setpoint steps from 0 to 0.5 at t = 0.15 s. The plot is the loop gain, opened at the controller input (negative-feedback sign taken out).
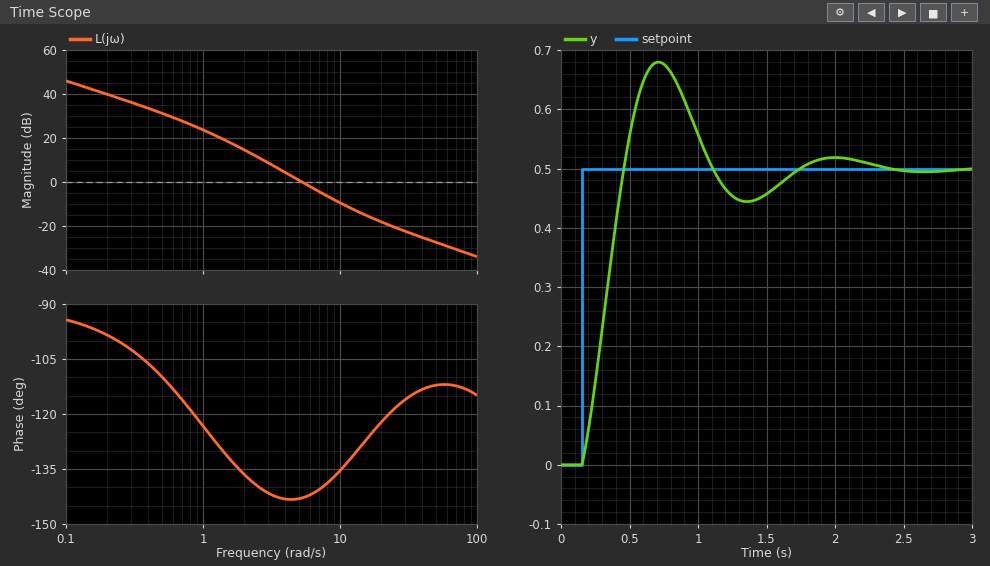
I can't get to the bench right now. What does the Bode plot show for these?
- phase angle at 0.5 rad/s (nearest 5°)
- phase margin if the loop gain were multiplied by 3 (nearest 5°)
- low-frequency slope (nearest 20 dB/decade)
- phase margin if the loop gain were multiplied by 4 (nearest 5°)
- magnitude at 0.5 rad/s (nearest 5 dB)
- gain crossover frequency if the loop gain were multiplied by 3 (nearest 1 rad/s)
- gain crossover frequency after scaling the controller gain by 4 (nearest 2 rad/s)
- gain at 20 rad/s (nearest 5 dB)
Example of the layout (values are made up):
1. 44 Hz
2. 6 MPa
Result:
1. -110°
2. 45°
3. -20 dB/decade
4. 50°
5. 30 dB
6. 10 rad/s
7. 12 rad/s
8. -20 dB
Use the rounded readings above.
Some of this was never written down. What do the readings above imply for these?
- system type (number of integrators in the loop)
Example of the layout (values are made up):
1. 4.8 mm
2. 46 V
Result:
1. 1
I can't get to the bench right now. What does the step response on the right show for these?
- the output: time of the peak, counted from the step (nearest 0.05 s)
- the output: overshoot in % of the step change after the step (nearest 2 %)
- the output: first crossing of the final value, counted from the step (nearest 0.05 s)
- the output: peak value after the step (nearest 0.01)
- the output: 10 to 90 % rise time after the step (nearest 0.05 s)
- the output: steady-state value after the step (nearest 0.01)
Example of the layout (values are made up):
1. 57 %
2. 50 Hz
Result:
1. 0.55 s
2. 36 %
3. 0.30 s
4. 0.68
5. 0.25 s
6. 0.50
